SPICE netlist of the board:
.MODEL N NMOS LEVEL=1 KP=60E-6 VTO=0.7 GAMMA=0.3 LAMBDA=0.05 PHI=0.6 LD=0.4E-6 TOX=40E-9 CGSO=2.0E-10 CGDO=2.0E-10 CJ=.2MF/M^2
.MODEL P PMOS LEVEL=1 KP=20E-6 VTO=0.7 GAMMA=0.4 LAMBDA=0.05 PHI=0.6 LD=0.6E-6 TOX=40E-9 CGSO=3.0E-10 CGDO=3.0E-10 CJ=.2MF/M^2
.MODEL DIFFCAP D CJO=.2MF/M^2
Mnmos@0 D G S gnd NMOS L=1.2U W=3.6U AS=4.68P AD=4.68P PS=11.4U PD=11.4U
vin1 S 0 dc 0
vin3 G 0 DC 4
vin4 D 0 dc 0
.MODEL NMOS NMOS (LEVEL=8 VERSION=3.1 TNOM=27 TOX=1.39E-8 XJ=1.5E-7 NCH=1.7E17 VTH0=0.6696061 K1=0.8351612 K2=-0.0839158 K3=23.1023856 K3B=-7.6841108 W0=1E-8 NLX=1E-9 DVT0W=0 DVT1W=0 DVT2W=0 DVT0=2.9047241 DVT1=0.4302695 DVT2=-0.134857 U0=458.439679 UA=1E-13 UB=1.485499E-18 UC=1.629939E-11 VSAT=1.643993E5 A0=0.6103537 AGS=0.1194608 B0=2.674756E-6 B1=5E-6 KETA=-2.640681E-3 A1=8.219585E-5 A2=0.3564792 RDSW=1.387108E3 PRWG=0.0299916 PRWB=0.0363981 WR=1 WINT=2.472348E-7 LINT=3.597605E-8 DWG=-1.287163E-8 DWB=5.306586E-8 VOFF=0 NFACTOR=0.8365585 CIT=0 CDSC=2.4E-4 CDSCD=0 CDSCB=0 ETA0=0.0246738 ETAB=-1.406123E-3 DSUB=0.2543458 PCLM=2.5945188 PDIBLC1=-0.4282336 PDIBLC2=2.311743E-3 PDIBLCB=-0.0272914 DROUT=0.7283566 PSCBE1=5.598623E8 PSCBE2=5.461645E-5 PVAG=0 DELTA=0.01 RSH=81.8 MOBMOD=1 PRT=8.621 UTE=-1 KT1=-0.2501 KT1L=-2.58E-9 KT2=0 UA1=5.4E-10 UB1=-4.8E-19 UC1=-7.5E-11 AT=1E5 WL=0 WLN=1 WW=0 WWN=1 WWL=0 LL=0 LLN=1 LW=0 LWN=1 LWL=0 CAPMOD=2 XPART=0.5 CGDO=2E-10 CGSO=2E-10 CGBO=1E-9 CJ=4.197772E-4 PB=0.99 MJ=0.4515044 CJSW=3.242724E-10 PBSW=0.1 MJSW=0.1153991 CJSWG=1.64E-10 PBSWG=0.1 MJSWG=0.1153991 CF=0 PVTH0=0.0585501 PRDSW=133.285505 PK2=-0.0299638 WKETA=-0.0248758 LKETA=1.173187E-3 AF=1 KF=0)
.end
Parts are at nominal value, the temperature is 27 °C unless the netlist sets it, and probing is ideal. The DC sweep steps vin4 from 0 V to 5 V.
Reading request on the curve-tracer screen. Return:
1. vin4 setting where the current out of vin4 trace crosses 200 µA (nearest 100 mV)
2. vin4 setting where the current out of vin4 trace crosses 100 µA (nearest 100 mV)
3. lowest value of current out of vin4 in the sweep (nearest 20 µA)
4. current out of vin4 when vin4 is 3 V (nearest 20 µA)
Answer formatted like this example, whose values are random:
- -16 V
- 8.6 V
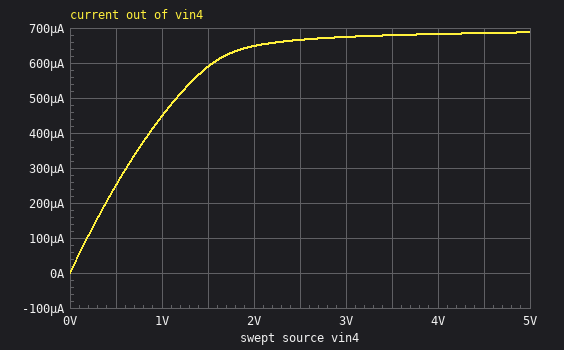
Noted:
- 400 mV
- 200 mV
- 0 A
- 680 µA
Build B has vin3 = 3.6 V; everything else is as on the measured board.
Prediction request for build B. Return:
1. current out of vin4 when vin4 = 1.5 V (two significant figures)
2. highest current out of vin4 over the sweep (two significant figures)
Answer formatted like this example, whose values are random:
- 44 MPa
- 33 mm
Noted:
- 510 µA
- 570 µA
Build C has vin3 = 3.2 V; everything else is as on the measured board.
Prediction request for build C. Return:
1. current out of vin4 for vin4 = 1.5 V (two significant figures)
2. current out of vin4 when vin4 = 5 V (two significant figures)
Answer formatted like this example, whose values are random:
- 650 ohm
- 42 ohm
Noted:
- 420 µA
- 460 µA
